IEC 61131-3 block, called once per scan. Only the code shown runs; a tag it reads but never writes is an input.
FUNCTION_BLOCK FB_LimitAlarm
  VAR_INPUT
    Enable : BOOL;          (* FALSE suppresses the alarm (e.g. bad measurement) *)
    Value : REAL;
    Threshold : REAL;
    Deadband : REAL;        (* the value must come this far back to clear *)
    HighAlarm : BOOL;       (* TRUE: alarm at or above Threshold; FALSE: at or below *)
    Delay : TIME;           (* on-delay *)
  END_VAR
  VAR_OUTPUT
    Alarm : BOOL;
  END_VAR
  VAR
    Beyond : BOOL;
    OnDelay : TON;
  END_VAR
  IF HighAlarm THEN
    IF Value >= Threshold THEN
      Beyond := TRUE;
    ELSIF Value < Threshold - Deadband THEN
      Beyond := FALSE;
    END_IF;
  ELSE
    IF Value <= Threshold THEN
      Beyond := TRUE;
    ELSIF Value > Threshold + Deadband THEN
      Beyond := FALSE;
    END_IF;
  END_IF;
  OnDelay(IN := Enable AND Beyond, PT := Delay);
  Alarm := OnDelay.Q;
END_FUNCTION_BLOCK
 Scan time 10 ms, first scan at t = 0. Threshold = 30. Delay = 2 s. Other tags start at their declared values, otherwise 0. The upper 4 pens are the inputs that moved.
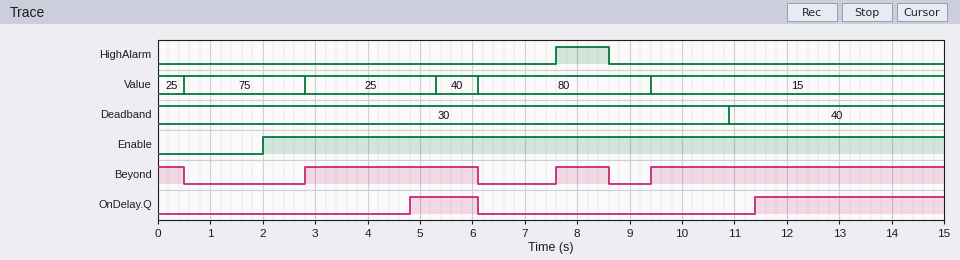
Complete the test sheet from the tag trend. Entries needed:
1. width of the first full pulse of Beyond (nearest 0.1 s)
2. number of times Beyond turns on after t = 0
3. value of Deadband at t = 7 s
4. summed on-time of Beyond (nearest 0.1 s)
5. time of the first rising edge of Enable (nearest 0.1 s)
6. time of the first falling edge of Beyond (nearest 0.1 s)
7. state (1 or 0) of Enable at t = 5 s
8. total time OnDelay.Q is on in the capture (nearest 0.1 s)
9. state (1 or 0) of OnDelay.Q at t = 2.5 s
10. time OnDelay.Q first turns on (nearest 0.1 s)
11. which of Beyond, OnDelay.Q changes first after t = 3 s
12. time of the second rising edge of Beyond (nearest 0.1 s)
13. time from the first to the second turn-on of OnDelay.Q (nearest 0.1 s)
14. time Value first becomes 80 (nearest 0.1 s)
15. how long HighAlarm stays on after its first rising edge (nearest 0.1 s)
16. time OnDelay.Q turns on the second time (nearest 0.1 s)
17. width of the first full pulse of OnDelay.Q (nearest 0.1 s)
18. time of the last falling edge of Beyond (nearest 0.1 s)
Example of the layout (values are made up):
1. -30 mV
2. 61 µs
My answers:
1. 3.3 s
2. 3
3. 30
4. 10.4 s
5. 2.0 s
6. 0.5 s
7. 1
8. 4.9 s
9. 0
10. 4.8 s
11. OnDelay.Q
12. 7.6 s
13. 6.6 s
14. 6.1 s
15. 1.0 s
16. 11.4 s
17. 1.3 s
18. 8.6 s
